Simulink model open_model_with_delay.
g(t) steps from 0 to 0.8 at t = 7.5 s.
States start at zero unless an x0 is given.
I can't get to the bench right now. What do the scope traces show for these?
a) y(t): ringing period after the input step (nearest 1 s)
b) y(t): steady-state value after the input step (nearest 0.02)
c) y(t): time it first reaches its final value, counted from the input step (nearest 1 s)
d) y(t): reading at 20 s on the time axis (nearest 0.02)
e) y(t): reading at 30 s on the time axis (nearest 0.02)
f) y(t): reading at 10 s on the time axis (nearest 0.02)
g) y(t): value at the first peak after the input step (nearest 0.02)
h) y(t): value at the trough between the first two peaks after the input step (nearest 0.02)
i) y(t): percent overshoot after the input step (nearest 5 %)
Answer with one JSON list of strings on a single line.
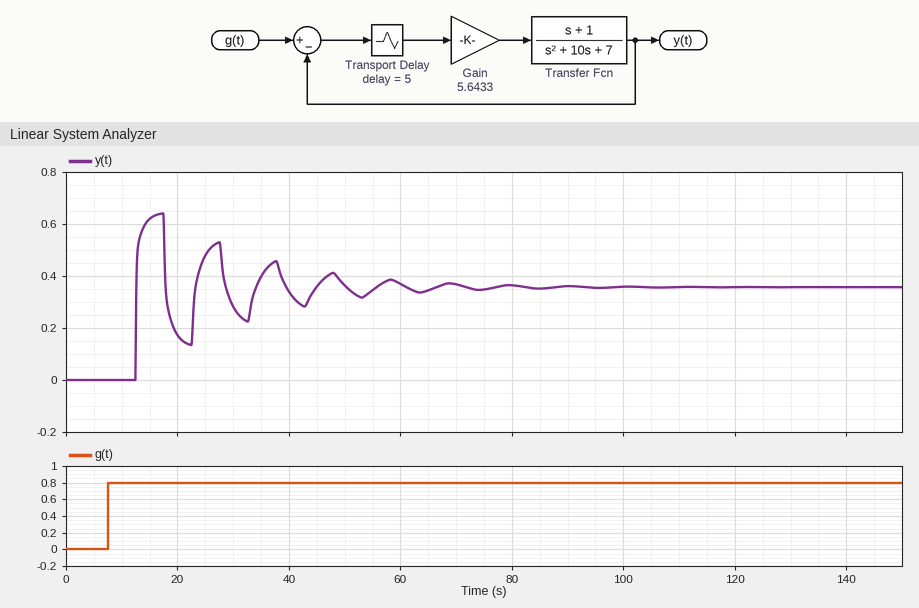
["10 s", "0.36", "5 s", "0.18", "0.28", "0.00", "0.64", "0.14", "80 %"]
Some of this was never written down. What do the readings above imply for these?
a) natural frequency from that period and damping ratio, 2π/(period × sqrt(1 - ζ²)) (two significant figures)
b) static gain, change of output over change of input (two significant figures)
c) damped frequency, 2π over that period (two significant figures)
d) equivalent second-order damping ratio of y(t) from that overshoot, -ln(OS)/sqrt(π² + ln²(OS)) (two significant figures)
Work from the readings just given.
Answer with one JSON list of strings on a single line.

["0.63 rad/s", "0.45", "0.63 rad/s", "0.071"]
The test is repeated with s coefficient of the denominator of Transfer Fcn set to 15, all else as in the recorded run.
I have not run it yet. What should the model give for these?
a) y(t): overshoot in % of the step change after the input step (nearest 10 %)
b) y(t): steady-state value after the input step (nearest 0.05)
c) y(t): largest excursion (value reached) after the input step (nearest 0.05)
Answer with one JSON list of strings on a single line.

["70 %", "0.35", "0.60"]
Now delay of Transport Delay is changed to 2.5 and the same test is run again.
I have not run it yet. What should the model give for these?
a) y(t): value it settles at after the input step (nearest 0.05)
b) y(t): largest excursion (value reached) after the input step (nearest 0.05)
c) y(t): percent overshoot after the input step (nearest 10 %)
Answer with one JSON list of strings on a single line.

["0.35", "0.60", "70 %"]
